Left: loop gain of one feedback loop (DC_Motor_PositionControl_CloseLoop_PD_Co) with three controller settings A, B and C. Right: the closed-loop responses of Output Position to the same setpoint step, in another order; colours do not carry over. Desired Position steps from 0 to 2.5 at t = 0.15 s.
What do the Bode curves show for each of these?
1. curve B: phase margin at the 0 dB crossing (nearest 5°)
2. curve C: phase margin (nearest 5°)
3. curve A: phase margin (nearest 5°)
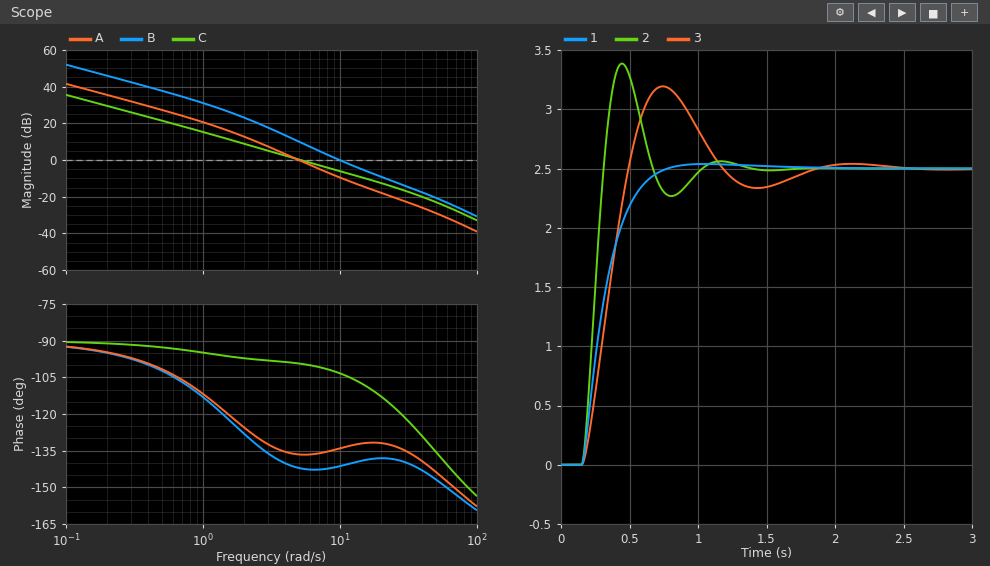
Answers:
40°
80°
45°
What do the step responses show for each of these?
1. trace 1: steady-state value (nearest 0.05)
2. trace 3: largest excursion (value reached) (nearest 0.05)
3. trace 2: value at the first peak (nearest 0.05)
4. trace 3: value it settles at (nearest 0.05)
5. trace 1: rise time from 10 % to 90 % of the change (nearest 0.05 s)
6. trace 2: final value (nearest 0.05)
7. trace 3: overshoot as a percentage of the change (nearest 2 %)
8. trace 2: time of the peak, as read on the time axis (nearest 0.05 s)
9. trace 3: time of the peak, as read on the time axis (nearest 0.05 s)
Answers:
2.50
3.20
3.40
2.50
0.35 s
2.50
28 %
0.45 s
0.75 s
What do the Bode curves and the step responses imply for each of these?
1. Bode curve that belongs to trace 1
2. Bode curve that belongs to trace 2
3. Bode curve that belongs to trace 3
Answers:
C
B
A
